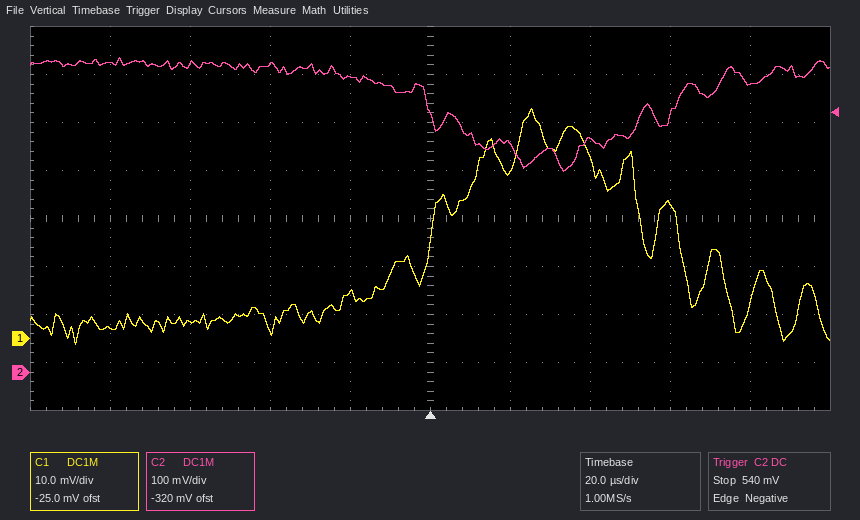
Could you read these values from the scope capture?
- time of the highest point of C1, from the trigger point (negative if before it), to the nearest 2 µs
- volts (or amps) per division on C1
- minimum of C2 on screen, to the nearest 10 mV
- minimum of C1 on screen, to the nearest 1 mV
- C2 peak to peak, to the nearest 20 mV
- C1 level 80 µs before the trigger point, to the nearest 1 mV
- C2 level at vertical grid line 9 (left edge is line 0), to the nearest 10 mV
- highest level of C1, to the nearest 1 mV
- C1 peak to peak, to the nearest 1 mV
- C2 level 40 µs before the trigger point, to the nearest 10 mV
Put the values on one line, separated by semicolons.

+26 µs; 10 mV; 420 mV; -1 mV; 240 mV; 2 mV; 600 mV; 48 mV; 49 mV; 640 mV
